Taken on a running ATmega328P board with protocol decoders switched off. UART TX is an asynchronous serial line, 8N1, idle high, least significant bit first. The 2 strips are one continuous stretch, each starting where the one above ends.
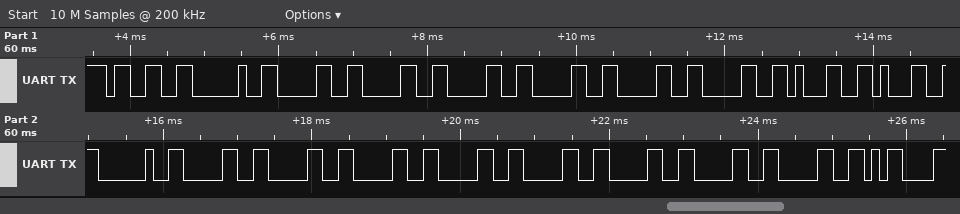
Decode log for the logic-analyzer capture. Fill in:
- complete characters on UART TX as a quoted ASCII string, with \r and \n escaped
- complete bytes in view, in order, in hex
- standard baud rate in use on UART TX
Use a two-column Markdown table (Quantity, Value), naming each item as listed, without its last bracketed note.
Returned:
| Quantity | Value |
|---|---|
| complete characters on UART TX as a quoted ASCII string, with \r and \n escaped | "3 00000011 00000000\r" |
| complete bytes in view, in order, in hex | 33 20 30 30 30 30 30 30 31 31 20 30 30 30 30 30 30 30 30 0D |
| standard baud rate in use on UART TX | 9600 baud |
